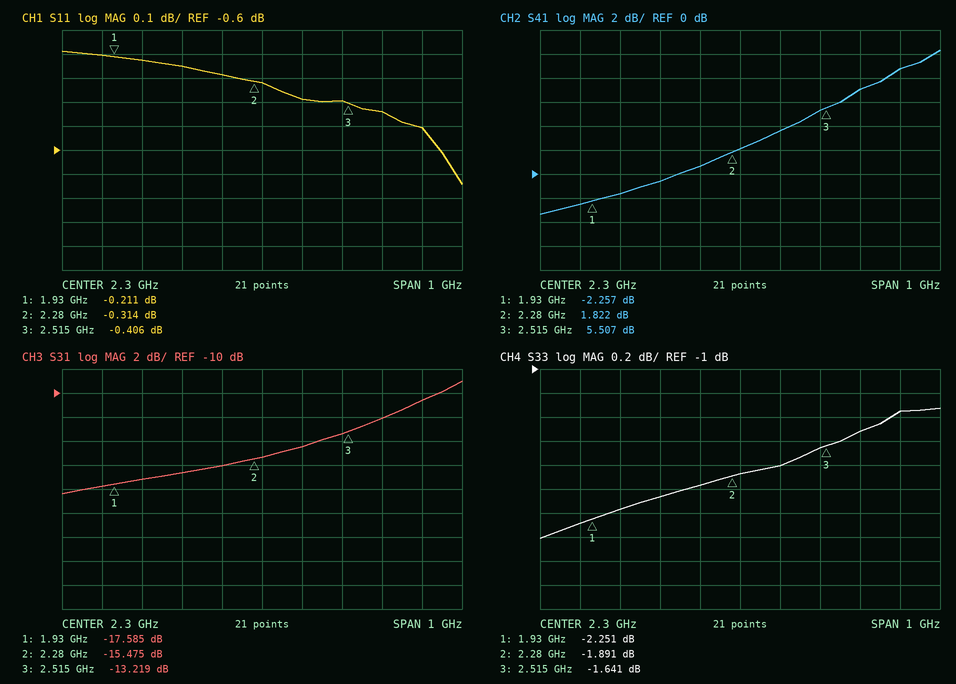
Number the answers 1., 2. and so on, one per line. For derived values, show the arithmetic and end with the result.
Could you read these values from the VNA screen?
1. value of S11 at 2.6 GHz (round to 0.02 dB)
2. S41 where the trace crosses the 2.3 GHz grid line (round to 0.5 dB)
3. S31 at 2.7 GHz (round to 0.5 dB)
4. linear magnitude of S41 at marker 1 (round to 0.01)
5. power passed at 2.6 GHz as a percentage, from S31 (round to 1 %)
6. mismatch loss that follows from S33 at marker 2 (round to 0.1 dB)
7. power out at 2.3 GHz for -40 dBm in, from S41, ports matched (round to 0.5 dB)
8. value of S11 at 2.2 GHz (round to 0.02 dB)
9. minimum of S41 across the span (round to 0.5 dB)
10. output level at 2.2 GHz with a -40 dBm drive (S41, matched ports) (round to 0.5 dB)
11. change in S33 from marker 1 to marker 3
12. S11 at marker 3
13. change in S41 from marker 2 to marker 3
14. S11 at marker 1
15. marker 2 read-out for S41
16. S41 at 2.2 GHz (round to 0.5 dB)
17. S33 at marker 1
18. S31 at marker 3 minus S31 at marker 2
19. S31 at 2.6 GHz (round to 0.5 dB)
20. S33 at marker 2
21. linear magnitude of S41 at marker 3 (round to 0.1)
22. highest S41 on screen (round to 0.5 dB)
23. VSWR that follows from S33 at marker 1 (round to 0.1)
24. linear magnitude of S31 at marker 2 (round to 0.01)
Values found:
1. -0.44 dB
2. 2.0 dB
3. -10.5 dB
4. 10^(-2.257/20) ≈ 0.77
5. 10^(-12/10) ≈ 6 %
6. −10 log10(1 − 10^(-1.891/10)) ≈ 4.5 dB
7. -40 dBm + (2.0 dB) = -38.0 dBm
8. -0.28 dB
9. -3.5 dB
10. -40 dBm + (0.5 dB) = -39.5 dBm
11. -1.641 − (-2.251) = 0.610 dB
12. -0.406 dB
13. 5.507 − (1.822) = 3.685 dB
14. -0.211 dB
15. 1.822 dB
16. 0.5 dB
17. -2.251 dB
18. -13.219 − (-15.475) = 2.256 dB
19. -12.0 dB
20. -1.891 dB
21. 10^(5.507/20) ≈ 1.9
22. 10.5 dB
23. (1 + 0.7717)/(1 − 0.7717) ≈ 7.8
24. 10^(-15.475/20) ≈ 0.17
